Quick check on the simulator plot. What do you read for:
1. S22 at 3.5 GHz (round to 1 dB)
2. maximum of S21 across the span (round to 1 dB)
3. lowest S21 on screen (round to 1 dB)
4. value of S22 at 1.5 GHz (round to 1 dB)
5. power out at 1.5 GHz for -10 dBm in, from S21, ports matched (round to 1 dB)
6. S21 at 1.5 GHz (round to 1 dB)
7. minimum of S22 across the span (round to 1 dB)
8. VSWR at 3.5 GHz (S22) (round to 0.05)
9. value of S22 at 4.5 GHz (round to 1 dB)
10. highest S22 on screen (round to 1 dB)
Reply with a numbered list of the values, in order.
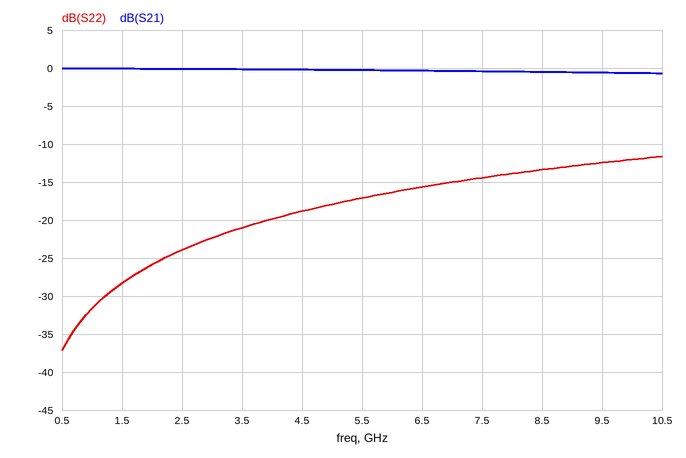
1. -21 dB
2. 0 dB
3. -1 dB
4. -28 dB
5. -10 dBm
6. 0 dB
7. -37 dB
8. 1.20
9. -19 dB
10. -12 dB
